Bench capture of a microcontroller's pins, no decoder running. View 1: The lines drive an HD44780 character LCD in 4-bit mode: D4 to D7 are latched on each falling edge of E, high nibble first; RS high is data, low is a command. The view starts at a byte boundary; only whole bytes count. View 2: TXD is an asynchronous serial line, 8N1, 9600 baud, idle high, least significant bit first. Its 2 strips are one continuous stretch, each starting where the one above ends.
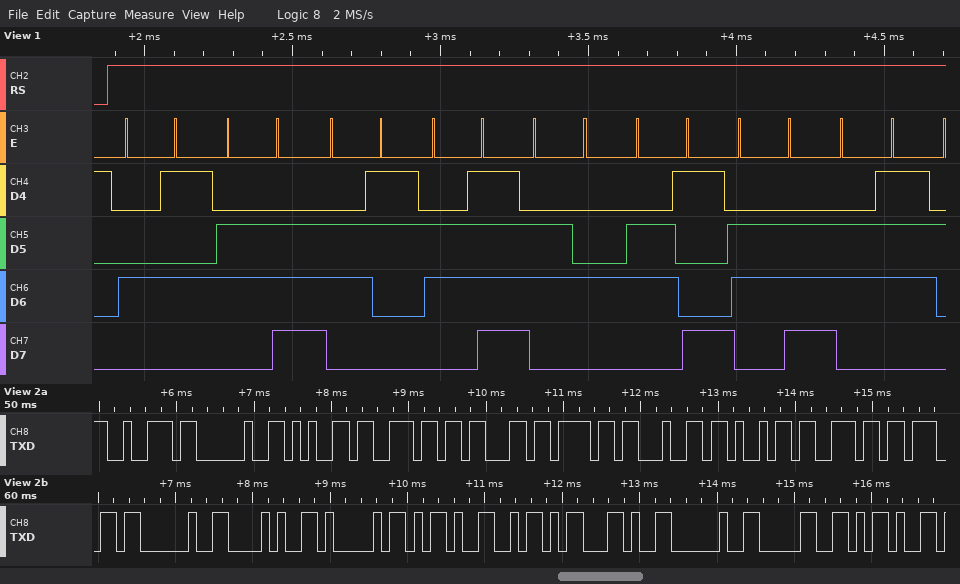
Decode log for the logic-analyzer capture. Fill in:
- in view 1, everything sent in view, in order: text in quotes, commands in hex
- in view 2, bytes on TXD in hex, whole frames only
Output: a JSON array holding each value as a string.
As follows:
["\"Encoding\"", "72 20 65 6E 63 6F 64 69 6E 67 20 28 41 2D 5A 2C 20 30 2D"]
